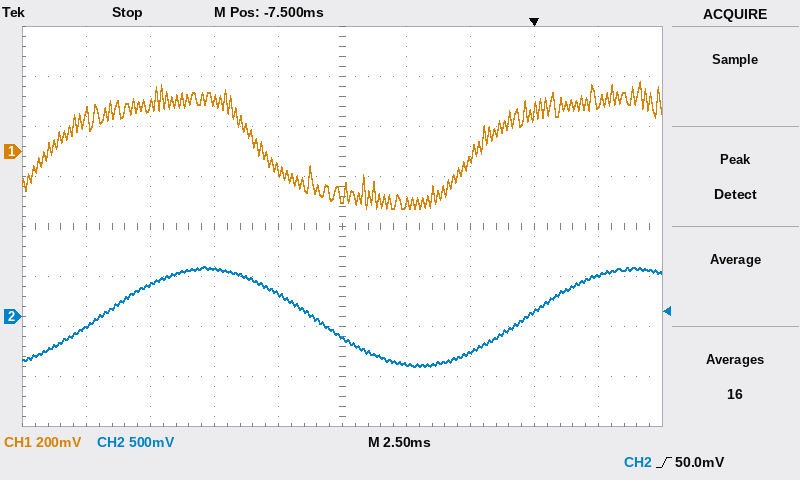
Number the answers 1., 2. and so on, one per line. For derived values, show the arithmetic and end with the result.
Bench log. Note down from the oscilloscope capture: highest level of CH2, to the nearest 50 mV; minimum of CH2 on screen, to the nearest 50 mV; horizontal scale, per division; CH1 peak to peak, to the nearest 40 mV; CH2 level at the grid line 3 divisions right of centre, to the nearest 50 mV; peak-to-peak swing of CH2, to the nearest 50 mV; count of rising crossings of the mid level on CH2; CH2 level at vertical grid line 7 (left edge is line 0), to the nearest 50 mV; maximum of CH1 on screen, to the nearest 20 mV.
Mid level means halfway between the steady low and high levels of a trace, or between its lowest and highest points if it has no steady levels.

1. 500 mV
2. -500 mV
3. 2.5 ms
4. 520 mV
5. 50 mV
6. 500 mV − (-500 mV) = 1.00 V
7. 2
8. -350 mV
9. 280 mV
